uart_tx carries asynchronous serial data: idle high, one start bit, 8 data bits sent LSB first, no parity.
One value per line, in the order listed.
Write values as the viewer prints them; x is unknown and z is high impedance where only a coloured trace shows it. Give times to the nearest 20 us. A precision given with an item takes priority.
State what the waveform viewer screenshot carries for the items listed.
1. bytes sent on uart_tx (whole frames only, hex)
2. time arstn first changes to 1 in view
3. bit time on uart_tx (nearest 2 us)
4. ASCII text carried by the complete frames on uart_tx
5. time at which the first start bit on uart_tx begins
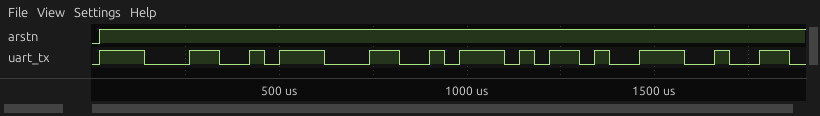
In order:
4C, 4C, 2D
20 us
40 us
"LL-"
140 us
